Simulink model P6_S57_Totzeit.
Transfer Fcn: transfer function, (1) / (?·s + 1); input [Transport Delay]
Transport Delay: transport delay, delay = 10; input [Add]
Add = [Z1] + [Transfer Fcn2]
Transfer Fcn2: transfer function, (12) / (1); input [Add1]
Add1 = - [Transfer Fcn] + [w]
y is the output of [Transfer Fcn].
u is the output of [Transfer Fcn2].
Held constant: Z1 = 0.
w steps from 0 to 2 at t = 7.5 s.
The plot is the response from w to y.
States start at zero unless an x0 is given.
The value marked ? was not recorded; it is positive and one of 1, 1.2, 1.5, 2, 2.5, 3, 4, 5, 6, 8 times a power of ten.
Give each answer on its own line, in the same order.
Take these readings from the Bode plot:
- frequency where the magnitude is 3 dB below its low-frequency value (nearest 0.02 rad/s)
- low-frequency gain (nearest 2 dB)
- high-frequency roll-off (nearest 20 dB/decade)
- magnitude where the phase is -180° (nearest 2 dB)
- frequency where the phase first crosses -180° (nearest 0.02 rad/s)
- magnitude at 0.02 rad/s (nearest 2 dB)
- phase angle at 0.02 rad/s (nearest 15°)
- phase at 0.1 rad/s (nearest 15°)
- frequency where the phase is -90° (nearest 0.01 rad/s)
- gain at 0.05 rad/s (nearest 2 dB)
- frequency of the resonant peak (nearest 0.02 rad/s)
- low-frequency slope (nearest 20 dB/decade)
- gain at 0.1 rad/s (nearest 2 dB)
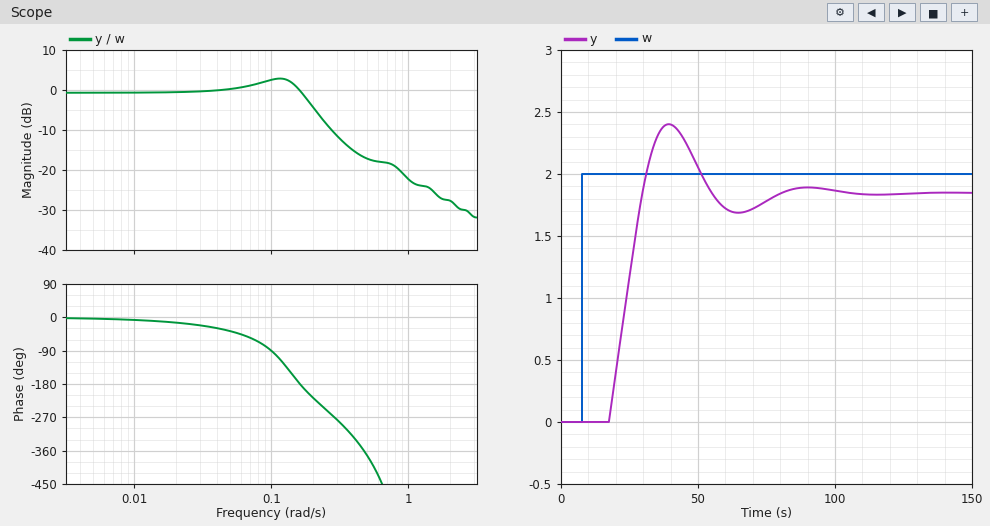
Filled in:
0.20 rad/s
0 dB
-20 dB/decade
0 dB
0.16 rad/s
0 dB
-15°
-90°
0.10 rad/s
0 dB
0.12 rad/s
0 dB/decade
2 dB
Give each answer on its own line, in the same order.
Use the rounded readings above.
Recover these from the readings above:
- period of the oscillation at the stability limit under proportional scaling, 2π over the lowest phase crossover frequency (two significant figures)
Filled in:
39 s
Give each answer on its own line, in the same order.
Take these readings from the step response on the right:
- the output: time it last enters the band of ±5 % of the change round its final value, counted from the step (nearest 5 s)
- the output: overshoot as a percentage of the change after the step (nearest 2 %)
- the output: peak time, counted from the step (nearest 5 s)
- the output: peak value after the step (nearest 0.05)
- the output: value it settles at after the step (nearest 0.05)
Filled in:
65 s
30 %
30 s
2.40
1.85
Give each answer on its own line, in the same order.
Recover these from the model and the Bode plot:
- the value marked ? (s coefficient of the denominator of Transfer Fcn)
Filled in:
150
